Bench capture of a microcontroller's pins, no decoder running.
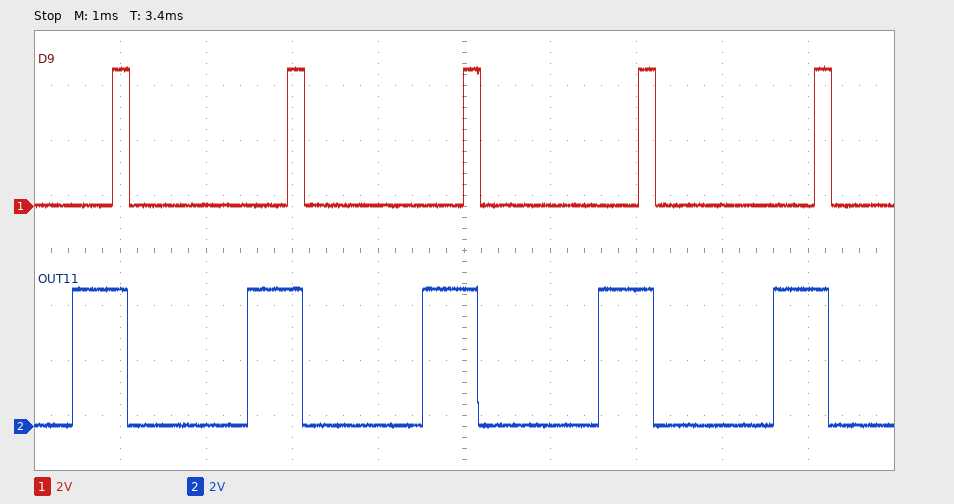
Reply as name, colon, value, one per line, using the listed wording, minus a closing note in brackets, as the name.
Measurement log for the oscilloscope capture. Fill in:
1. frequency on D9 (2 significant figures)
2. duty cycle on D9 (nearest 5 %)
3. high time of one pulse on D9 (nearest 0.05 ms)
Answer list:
frequency on D9: 490 Hz
duty cycle on D9: 10 %
high time of one pulse on D9: 0.20 ms
